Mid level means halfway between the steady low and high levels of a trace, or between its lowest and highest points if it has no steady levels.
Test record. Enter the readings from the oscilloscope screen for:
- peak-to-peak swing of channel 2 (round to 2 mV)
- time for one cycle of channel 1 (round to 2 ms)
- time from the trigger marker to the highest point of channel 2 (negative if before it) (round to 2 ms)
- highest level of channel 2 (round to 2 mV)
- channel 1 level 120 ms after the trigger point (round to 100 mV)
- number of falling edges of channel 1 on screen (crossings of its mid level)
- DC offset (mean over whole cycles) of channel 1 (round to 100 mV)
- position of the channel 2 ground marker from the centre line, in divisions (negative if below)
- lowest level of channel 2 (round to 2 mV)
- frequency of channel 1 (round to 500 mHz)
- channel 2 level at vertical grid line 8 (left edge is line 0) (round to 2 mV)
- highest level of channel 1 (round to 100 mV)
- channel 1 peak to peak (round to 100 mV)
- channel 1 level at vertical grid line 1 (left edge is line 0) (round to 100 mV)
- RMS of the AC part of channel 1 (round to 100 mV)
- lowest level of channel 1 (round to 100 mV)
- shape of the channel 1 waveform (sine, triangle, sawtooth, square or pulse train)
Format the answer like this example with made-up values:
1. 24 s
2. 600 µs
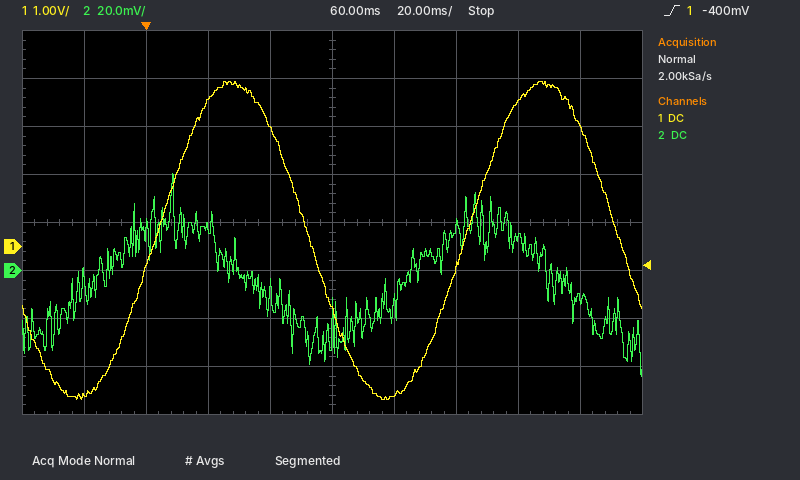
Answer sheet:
1. 84 mV
2. 100 ms
3. +8 ms
4. 40 mV
5. 3.0 V
6. 2
7. 100 mV
8. -1.0 div
9. -44 mV
10. 10.0 Hz
11. 14 mV
12. 3.4 V
13. 6.6 V
14. -3.1 V
15. 2.3 V
16. -3.2 V
17. sine
